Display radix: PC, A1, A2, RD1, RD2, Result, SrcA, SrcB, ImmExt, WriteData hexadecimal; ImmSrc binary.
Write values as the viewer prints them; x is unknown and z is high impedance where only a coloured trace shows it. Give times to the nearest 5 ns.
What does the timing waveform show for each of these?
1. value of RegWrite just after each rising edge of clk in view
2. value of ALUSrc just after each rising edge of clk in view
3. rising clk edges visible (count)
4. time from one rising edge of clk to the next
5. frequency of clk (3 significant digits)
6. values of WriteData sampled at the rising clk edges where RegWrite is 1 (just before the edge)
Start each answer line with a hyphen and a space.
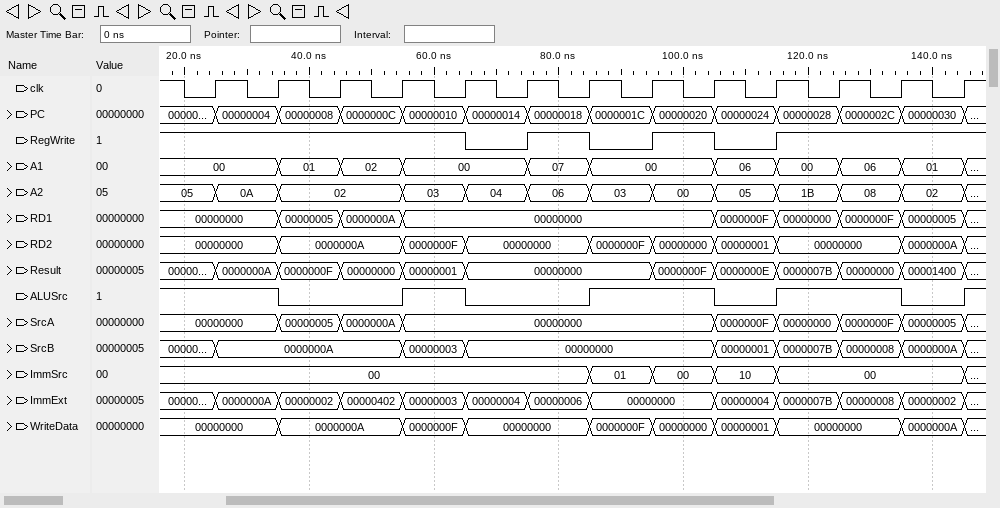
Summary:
- 1 1 1 1 0 1 0 1 0 1 1 1 1
- 1 0 0 1 0 0 1 1 0 1 1 0 1
- 13
- 10 ns
- 100 MHz
- 00000000, 00000000, 0000000A, 0000000A, 0000000F, 00000000, 00000000, 00000000, 00000000, 0000000A
